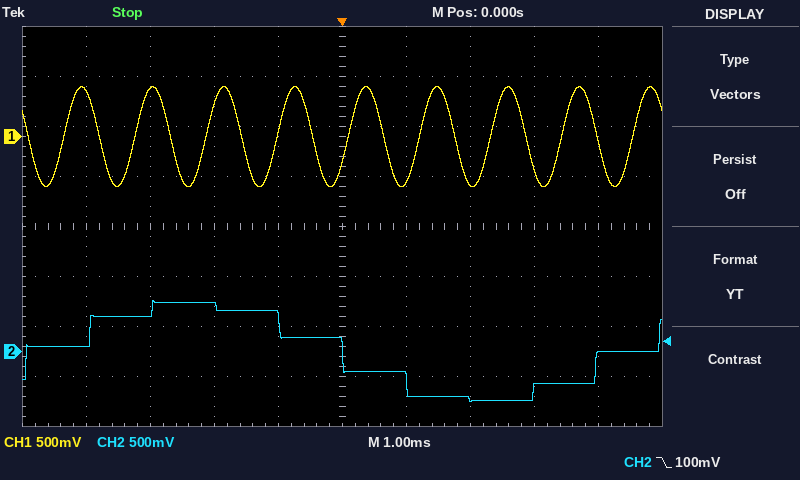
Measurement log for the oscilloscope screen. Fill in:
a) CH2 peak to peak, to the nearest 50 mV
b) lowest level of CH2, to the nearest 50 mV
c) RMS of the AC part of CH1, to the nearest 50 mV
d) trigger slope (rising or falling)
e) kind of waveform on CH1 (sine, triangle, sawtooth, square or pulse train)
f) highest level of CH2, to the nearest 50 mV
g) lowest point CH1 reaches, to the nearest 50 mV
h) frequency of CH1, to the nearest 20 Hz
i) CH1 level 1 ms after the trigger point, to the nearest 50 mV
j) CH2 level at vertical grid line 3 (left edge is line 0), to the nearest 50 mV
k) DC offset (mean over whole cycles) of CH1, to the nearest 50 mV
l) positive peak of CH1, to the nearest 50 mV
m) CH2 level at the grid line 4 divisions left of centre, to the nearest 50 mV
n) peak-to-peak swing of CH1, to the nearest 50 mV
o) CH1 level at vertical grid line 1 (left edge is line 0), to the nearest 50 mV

1.00 V
-500 mV
350 mV
falling
sine
500 mV
-500 mV
900 Hz
-450 mV
450 mV
0 mV
500 mV
50 mV
1.00 V
450 mV
